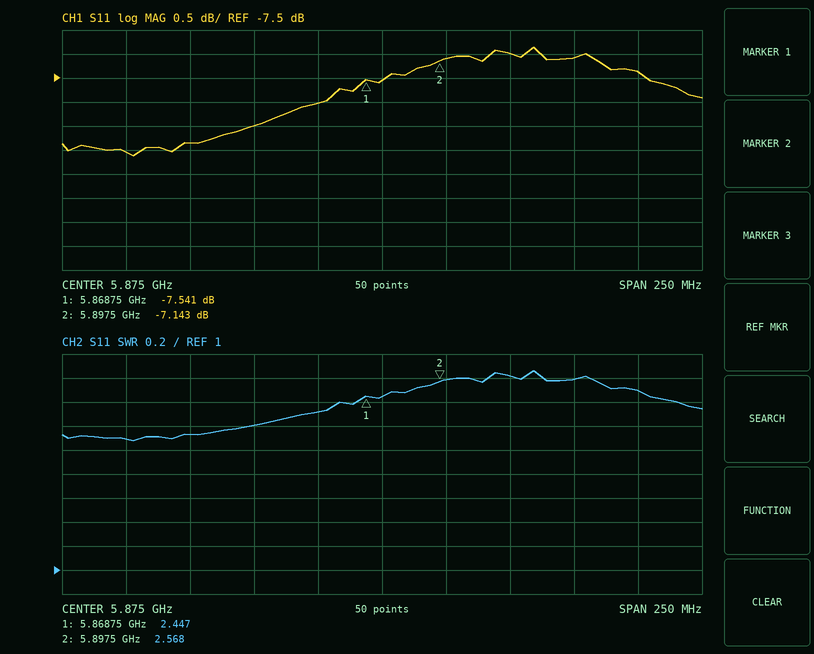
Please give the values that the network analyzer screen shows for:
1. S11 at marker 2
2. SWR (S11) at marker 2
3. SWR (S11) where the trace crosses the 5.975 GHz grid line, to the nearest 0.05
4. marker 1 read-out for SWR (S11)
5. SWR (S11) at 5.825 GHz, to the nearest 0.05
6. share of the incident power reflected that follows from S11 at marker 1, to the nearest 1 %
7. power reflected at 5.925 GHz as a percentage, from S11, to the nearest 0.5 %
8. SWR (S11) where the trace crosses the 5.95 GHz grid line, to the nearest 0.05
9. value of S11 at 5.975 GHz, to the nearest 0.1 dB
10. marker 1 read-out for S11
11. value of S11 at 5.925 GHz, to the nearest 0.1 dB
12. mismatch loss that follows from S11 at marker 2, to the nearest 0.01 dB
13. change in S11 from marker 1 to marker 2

-7.143 dB
2.568
2.50
2.447
2.20
18 %
20.0 %
2.60
-7.4 dB
-7.541 dB
-7.0 dB
0.93 dB
0.398 dB
